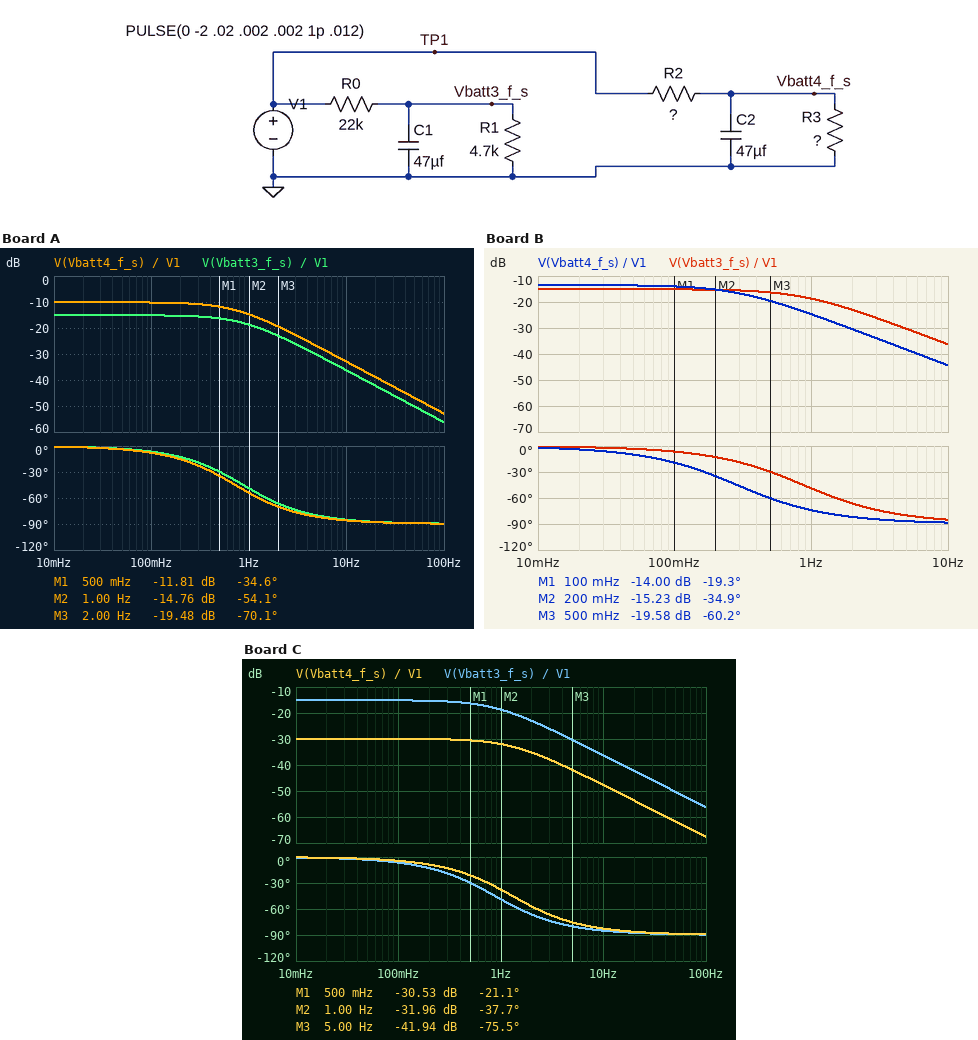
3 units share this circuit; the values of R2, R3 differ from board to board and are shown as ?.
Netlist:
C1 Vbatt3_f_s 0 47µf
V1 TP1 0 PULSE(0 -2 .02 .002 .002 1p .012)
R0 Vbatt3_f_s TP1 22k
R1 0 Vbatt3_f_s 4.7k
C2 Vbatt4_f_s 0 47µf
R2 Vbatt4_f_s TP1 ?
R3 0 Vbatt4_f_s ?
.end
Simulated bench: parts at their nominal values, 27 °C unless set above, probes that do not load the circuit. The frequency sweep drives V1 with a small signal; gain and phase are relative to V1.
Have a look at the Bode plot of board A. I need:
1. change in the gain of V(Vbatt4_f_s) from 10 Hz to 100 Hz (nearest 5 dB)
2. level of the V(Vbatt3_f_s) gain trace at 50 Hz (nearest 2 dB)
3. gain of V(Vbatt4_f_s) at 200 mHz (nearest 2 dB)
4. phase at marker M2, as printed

-20 dB
-50 dB
-10 dB
-54.1 deg
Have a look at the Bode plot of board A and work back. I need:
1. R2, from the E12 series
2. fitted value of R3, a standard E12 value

15 kΩ
6.8 kΩ
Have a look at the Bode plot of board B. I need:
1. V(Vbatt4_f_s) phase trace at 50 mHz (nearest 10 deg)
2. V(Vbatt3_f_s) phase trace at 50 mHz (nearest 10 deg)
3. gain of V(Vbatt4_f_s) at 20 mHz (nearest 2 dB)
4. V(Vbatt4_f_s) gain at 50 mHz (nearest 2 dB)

-10 deg
0 deg
-14 dB
-14 dB
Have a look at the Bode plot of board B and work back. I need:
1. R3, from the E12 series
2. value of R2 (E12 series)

15 kΩ
56 kΩ
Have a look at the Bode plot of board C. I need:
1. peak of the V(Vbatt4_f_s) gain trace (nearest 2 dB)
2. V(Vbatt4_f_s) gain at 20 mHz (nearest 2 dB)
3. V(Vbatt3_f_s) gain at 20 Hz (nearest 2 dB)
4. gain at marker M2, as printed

-30 dB
-30 dB
-42 dB
-31.96 dB
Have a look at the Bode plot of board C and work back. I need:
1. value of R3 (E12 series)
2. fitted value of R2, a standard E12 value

2.7 kΩ
82 kΩ
